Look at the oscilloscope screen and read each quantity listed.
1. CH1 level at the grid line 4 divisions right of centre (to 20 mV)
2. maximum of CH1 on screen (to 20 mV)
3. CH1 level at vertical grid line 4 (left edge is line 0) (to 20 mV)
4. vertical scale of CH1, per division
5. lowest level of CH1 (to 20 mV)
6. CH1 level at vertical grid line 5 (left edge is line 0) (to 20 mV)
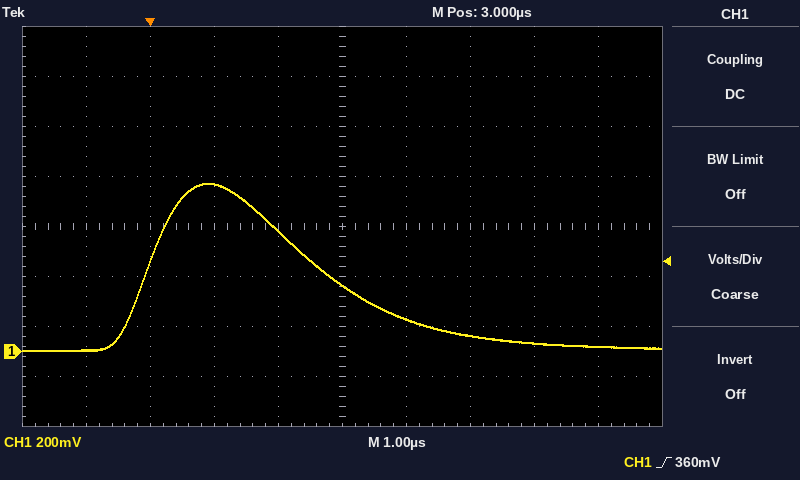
20 mV
680 mV
480 mV
200 mV
0 mV
260 mV
